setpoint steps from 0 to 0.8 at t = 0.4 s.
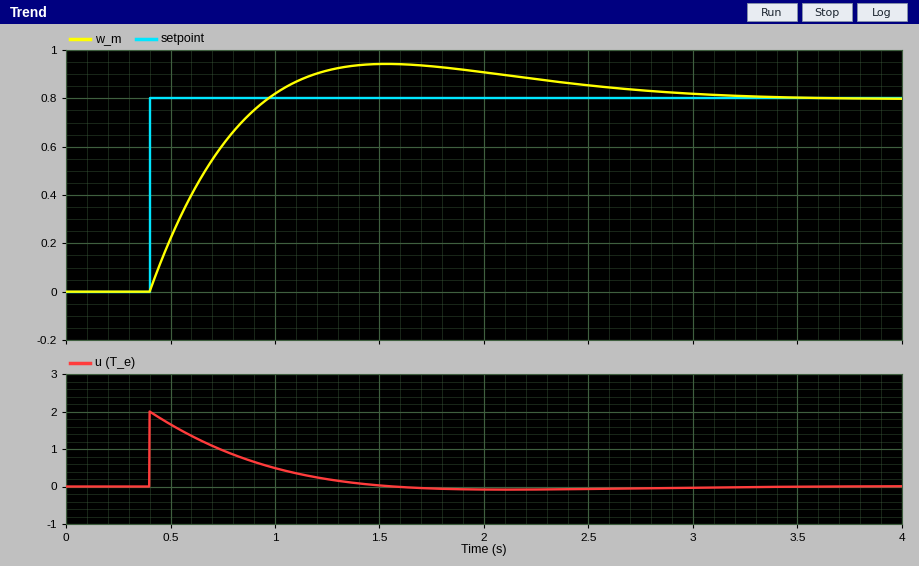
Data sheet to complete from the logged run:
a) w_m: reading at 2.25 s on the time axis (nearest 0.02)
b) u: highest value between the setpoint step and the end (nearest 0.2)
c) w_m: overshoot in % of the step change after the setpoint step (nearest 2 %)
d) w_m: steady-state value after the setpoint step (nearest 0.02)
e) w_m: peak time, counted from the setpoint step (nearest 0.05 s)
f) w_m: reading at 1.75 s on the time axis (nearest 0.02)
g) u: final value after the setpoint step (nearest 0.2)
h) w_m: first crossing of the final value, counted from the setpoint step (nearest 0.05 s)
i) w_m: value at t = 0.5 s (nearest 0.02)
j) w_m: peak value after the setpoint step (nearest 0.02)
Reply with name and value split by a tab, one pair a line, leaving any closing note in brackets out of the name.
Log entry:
w_m: reading at 2.25 s on the time axis	0.88
u: highest value between the setpoint step and the end	2.0
w_m: overshoot in % of the step change after the setpoint step	18 %
w_m: steady-state value after the setpoint step	0.80
w_m: peak time, counted from the setpoint step	1.15 s
w_m: reading at 1.75 s on the time axis	0.94
u: final value after the setpoint step	0.0
w_m: first crossing of the final value, counted from the setpoint step	0.55 s
w_m: value at t = 0.5 s	0.22
w_m: peak value after the setpoint step	0.94
